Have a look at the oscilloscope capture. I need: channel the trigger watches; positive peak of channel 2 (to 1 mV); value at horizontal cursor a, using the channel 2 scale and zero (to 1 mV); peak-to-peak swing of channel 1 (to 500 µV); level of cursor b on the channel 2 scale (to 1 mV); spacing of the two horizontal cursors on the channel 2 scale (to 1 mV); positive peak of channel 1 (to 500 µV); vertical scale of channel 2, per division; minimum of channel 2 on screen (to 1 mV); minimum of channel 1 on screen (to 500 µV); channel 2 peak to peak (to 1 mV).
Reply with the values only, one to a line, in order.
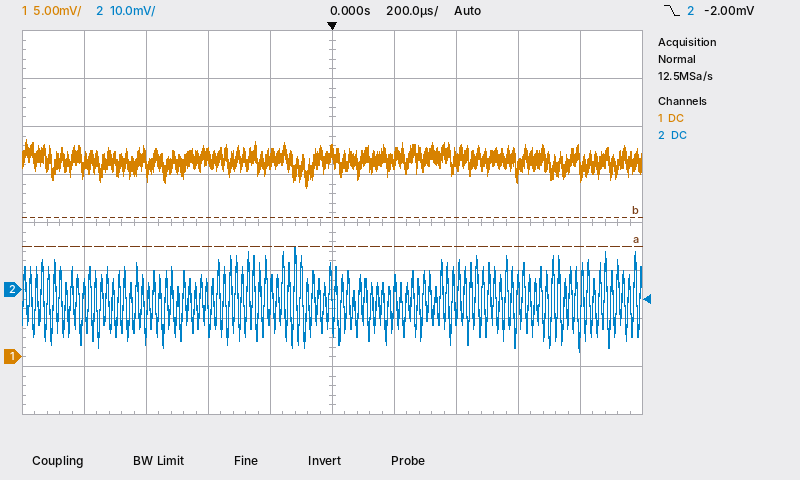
channel 2
9 mV
9 mV
5.0 mV
15 mV
6 mV
22.5 mV
10 mV
-13 mV
17.5 mV
22 mV
